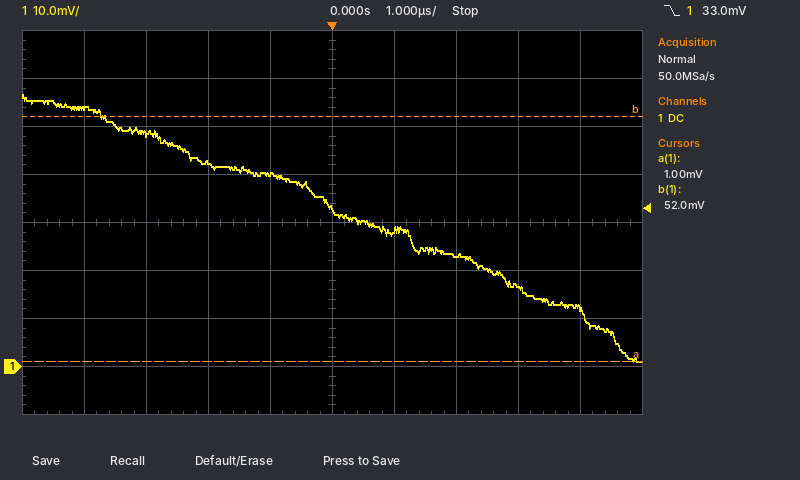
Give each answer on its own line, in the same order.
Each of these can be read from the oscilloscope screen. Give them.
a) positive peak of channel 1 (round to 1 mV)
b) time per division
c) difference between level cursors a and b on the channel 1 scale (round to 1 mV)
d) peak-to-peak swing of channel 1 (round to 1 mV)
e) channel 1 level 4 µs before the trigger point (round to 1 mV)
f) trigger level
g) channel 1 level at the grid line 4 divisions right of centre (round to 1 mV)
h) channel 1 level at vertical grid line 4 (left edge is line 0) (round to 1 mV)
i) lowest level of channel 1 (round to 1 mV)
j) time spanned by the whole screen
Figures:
57 mV
1 µs
51 mV
56 mV
54 mV
33.0 mV
12 mV
40 mV
1 mV
10 µs
